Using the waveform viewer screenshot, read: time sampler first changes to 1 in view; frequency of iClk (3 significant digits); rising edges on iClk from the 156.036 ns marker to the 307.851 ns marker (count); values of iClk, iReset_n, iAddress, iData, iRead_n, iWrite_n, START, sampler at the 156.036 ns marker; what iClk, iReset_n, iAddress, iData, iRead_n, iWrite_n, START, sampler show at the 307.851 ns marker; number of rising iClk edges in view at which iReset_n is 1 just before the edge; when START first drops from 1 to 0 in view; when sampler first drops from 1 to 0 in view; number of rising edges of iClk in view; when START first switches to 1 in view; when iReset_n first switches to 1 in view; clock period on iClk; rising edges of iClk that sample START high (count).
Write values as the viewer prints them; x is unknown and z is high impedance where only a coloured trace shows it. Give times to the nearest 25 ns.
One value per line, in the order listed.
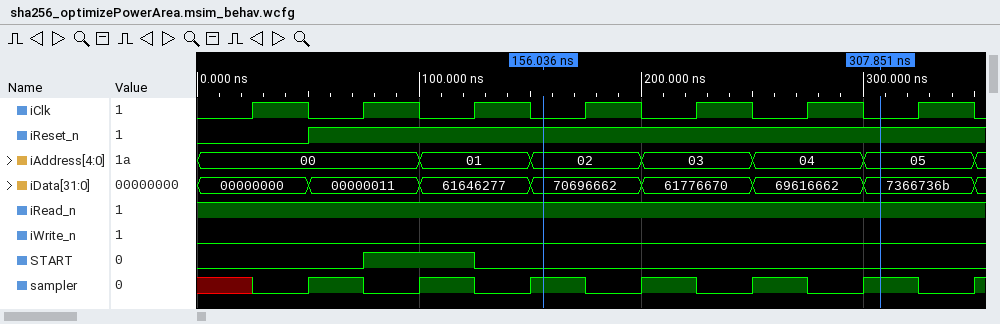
50 ns
20.0 MHz
3
iClk=0, iReset_n=1, iAddress=02, iData=70696662, iRead_n=1, iWrite_n=0, START=0, sampler=1
iClk=0, iReset_n=1, iAddress=05, iData=7366736b, iRead_n=1, iWrite_n=0, START=0, sampler=1
6
125 ns
75 ns
7
75 ns
50 ns
50 ns
1
